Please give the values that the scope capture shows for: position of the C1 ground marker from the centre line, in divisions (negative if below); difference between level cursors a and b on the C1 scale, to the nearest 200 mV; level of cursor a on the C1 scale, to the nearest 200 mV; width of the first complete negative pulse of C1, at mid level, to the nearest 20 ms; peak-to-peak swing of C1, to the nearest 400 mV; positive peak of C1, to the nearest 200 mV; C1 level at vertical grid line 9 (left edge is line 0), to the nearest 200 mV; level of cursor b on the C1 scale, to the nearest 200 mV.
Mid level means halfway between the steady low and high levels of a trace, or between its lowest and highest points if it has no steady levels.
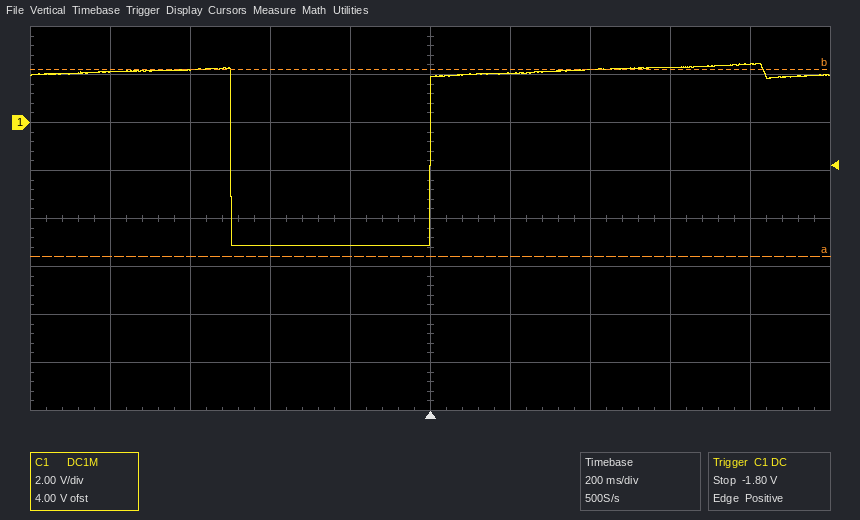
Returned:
+2.0 div
7.8 V
-5.6 V
500 ms
7.6 V
2.4 V
2.4 V
2.2 V
